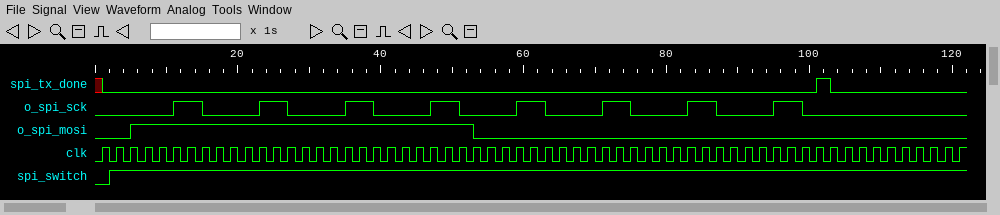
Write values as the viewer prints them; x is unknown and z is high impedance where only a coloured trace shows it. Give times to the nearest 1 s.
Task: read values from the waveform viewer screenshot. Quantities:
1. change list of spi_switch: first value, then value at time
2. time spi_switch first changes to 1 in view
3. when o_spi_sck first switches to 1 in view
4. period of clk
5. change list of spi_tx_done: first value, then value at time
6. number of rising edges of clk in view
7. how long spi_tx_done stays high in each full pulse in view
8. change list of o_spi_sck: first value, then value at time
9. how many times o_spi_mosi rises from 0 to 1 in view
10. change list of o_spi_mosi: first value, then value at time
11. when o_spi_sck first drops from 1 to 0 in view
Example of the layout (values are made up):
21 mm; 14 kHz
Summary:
0, 1 at 2 s; 2 s; 11 s; 2 s; x, 0 at 1 s, 1 at 101 s, 0 at 103 s; 61; 2 s; 0, 1 at 11 s, 0 at 15 s, 1 at 23 s, 0 at 27 s, 1 at 35 s, 0 at 39 s, 1 at 47 s, 0 at 51 s, 1 at 59 s, 0 at 63 s, 1 at 71 s, 0 at 75 s, 1 at 83 s, 0 at 87 s, 1 at 95 s, 0 at 99 s; 1; 0, 1 at 5 s, 0 at 53 s; 15 s
